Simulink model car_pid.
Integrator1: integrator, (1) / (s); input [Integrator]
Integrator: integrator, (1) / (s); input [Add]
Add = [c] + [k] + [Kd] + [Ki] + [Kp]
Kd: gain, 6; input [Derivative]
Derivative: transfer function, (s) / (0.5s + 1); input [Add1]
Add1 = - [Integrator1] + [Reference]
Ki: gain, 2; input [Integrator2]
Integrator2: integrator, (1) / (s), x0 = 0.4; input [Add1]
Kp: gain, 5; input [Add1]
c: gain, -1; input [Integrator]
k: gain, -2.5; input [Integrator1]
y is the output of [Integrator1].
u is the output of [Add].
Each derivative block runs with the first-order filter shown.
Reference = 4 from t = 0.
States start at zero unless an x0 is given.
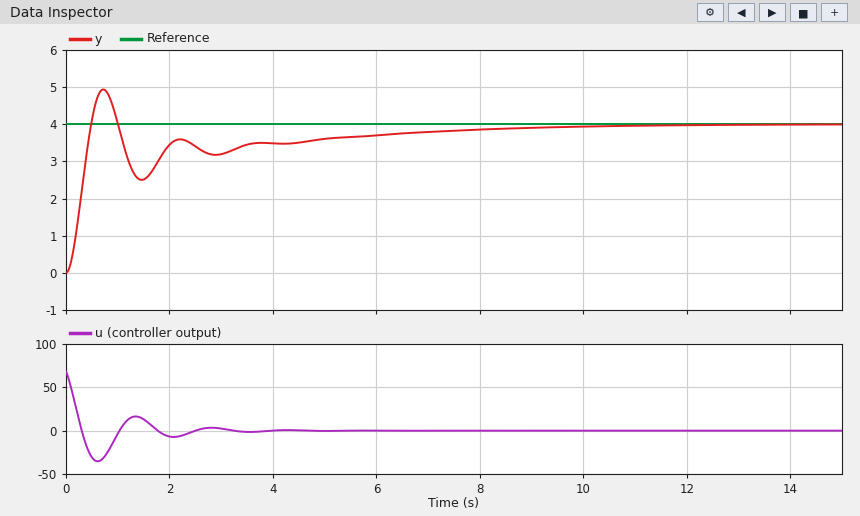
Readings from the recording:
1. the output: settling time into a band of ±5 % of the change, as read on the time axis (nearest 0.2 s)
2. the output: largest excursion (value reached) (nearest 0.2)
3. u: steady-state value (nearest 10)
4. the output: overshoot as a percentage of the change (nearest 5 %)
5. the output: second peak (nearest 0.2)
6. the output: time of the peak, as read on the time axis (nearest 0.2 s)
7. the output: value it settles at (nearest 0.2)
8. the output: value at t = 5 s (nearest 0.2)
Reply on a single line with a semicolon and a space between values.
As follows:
7.2 s; 5.0; 0; 25 %; 3.6; 0.8 s; 4.0; 3.6
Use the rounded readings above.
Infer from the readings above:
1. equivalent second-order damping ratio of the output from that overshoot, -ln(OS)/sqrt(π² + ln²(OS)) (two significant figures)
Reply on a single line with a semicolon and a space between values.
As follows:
0.40
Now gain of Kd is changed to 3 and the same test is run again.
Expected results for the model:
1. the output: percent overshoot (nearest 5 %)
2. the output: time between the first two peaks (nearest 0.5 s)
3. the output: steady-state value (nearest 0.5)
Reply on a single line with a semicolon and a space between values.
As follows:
20 %; 2.0 s; 4.0
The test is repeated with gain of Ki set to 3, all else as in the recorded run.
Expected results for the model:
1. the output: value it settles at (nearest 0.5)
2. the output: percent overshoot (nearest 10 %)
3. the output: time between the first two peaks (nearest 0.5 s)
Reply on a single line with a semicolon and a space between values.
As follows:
4.0; 30 %; 1.5 s
